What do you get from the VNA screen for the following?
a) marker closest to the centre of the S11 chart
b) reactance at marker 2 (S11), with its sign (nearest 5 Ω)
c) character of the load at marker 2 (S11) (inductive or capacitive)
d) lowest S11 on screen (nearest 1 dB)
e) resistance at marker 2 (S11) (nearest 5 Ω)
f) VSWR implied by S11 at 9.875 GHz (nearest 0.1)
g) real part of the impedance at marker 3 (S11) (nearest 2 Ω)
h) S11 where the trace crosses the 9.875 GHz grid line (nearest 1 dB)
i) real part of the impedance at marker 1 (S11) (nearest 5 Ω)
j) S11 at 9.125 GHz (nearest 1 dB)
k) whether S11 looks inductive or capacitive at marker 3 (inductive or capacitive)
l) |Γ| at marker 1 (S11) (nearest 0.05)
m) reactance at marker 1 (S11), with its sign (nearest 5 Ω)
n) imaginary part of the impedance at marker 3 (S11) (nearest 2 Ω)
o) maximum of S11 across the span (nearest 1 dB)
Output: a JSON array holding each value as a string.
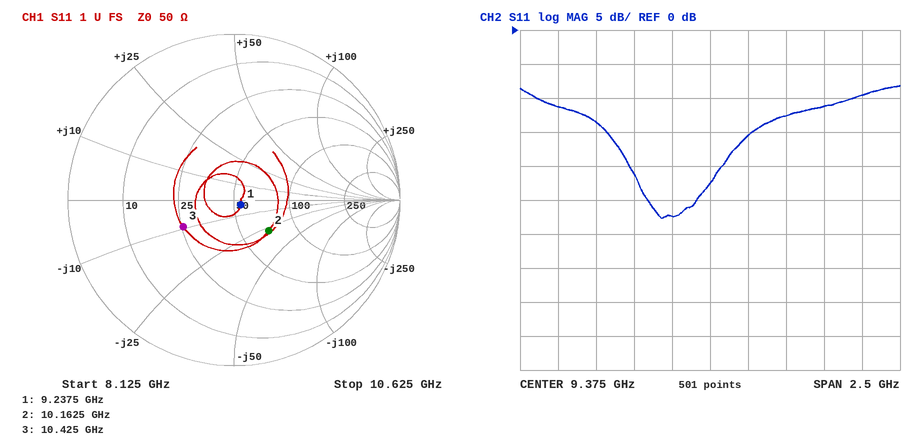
["marker 1", "-30 Ω", "capacitive", "-28 dB", "70 Ω", "1.6", "26 Ω", "-13 dB", "55 Ω", "-27 dB", "capacitive", "0.05", "-5 Ω", "-10 Ω", "-8 dB"]
